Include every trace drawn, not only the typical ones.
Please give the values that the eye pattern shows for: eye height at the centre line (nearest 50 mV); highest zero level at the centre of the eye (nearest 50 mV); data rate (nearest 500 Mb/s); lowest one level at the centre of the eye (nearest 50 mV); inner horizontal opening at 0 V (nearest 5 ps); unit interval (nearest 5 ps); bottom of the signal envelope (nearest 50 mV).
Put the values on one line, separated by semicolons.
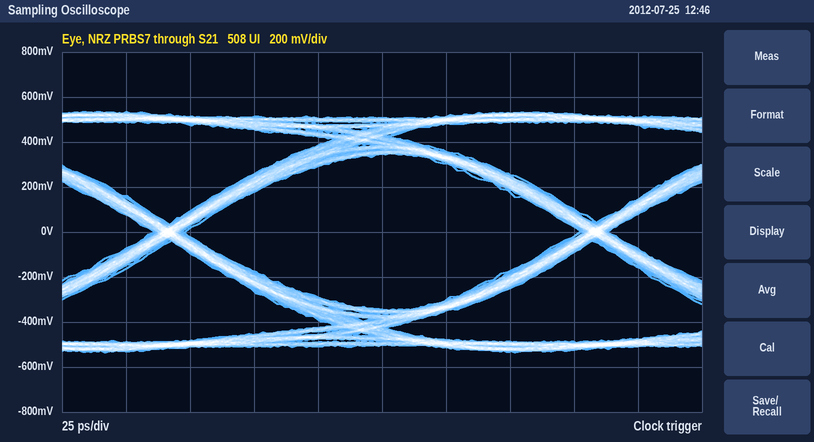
700 mV; -350 mV; 6.0 Gb/s; 350 mV; 155 ps; 165 ps; -550 mV
